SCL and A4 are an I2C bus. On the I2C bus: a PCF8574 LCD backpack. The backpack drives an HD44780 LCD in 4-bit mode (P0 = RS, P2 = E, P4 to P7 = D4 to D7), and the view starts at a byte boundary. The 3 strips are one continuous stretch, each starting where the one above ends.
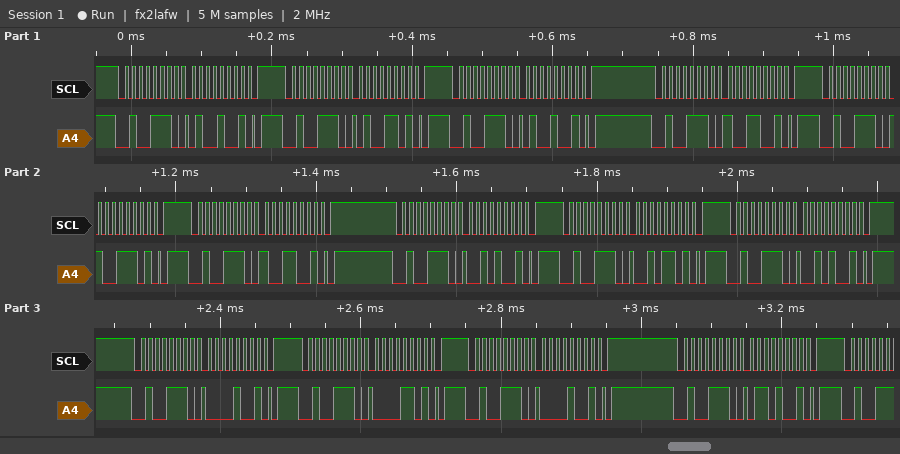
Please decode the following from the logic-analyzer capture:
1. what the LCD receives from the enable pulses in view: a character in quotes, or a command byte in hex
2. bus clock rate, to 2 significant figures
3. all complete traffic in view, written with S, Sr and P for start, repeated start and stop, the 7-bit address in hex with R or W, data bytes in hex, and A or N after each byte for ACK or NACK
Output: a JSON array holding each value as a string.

["'I' ' '", "100 kHz", "S 27W A 49 A P S 27W A 4D A P S 27W A 49 A P S 27W A 99 A P S 27W A 9D A P S 27W A 99 A P S 27W A 29 A P S 27W A 2D A P S 27W A 29 A P S 27W A 09 A P S 27W A 0D A P S 27W A 09 A P S 27W A 69 A P"]
